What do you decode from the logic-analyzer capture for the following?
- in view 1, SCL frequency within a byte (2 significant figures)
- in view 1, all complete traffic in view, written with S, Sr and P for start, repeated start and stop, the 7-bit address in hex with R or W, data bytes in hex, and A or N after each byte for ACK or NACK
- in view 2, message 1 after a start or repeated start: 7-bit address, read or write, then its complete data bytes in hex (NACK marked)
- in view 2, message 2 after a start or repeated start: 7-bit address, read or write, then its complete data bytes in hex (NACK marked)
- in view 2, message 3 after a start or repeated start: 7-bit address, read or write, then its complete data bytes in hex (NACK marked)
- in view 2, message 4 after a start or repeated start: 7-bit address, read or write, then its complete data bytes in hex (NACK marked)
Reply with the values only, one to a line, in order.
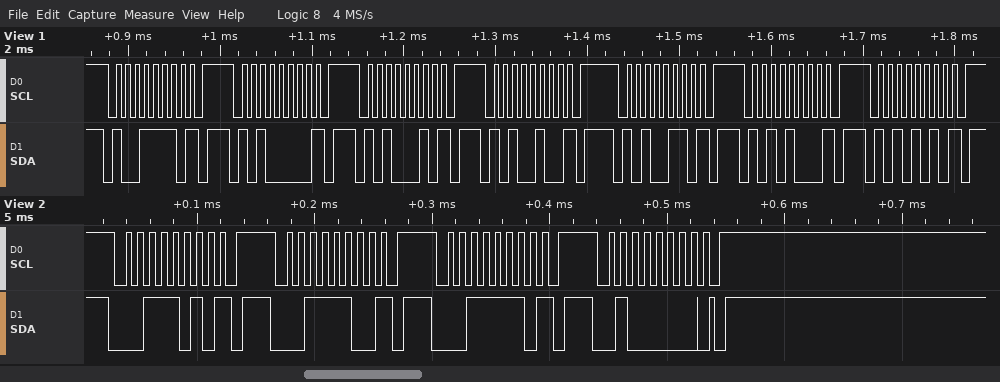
100 kHz
S 4FW N P S 50W N P S 51W N P S 52W N P S 53W N P S 54W N P S 55W N P
0x1D write NACK
0x1E write NACK
0x1F write NACK
0x20 write
